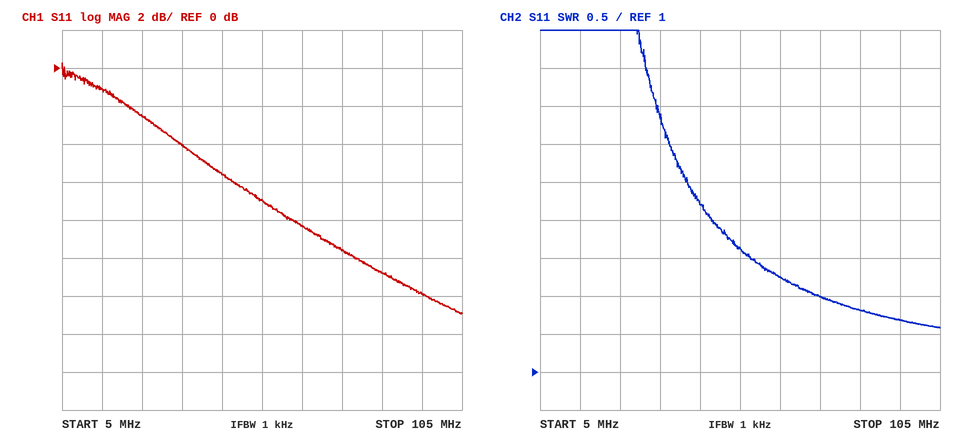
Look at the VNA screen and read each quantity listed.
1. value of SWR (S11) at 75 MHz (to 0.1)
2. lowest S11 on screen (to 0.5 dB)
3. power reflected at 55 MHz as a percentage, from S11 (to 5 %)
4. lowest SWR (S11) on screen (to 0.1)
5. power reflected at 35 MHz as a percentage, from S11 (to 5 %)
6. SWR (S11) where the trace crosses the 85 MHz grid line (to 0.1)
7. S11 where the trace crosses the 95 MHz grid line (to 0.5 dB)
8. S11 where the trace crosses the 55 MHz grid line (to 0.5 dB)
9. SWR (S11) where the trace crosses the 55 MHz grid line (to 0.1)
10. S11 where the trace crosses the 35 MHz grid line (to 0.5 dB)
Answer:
2.0
-13.0 dB
20 %
1.6
40 %
1.8
-12.0 dB
-7.0 dB
2.6
-4.0 dB
